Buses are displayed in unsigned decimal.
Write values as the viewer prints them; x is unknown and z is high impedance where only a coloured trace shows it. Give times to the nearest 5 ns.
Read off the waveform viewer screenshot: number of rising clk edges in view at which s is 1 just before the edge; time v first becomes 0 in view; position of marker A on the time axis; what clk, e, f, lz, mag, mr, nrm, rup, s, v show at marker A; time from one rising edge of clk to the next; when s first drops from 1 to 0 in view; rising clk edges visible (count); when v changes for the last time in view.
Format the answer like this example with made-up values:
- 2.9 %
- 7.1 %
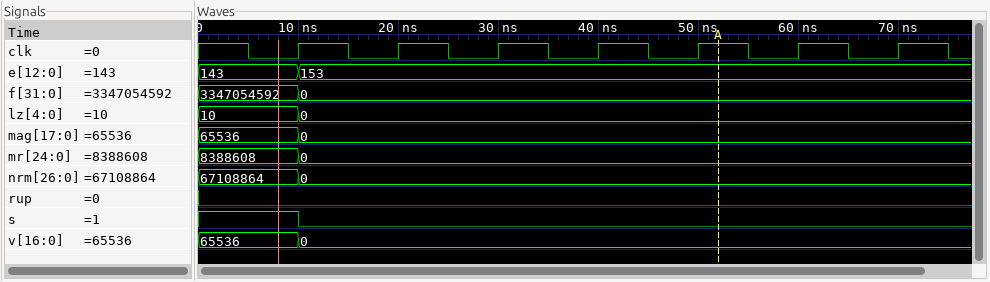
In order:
- 1
- 10 ns
- 50 ns
- clk=1, e=153, f=0, lz=0, mag=0, mr=0, nrm=0, rup=0, s=0, v=0
- 10 ns
- 10 ns
- 7
- 10 ns
